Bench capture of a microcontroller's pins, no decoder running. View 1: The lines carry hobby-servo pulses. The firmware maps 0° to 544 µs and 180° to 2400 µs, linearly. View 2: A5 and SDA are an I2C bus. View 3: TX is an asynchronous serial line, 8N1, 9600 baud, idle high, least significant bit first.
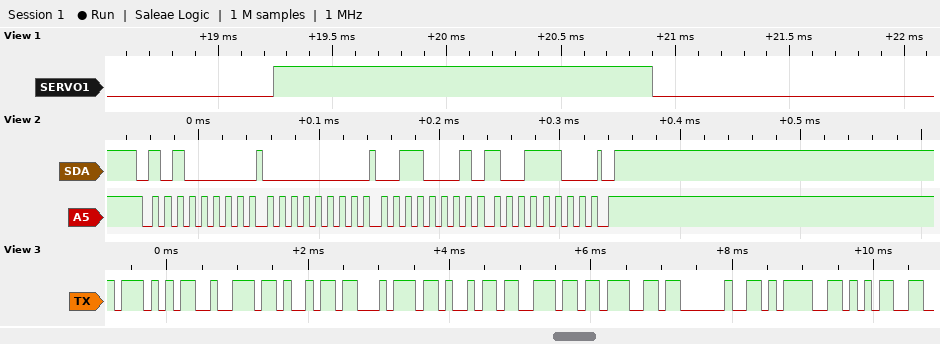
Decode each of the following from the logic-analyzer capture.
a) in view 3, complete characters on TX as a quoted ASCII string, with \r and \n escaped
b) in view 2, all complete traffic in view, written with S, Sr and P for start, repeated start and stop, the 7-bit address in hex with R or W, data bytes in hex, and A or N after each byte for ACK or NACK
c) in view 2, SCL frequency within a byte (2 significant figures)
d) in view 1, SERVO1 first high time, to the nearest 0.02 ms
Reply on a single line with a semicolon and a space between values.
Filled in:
"Writing =5"; S 50W A 00 A 31 A 9C A P; 100 kHz; 1.66 ms
